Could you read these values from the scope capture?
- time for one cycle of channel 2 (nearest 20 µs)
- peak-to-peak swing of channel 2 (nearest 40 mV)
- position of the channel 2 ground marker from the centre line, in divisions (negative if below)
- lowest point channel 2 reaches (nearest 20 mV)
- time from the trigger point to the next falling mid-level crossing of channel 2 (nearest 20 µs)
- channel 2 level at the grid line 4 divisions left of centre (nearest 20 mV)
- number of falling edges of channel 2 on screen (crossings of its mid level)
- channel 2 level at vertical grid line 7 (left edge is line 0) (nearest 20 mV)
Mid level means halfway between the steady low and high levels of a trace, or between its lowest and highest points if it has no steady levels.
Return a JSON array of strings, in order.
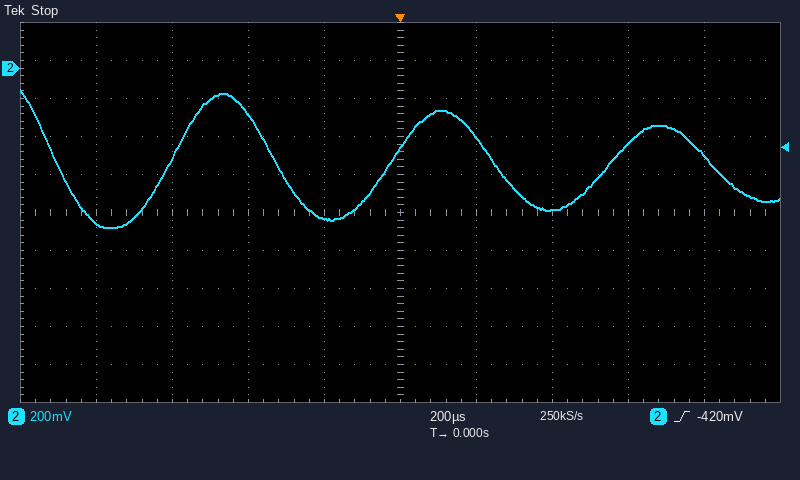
["580 µs", "720 mV", "+3.8 div", "-840 mV", "240 µs", "-820 mV", "4", "-740 mV"]
